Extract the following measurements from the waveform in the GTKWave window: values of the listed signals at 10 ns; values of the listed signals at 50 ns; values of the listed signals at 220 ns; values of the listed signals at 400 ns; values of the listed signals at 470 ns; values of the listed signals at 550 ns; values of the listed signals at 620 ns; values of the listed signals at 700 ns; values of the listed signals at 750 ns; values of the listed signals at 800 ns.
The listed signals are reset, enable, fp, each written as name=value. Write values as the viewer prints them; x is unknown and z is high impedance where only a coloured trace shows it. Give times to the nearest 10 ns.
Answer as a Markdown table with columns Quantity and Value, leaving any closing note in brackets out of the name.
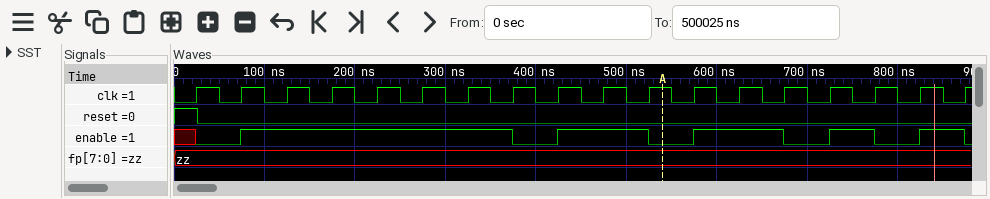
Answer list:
| Quantity | Value |
|---|---|
| values of the listed signals at 10 ns | reset=1, enable=x, fp=zz |
| values of the listed signals at 50 ns | reset=0, enable=0, fp=zz |
| values of the listed signals at 220 ns | reset=0, enable=1, fp=zz |
| values of the listed signals at 400 ns | reset=0, enable=0, fp=zz |
| values of the listed signals at 470 ns | reset=0, enable=1, fp=zz |
| values of the listed signals at 550 ns | reset=0, enable=0, fp=zz |
| values of the listed signals at 620 ns | reset=0, enable=1, fp=zz |
| values of the listed signals at 700 ns | reset=0, enable=0, fp=zz |
| values of the listed signals at 750 ns | reset=0, enable=1, fp=zz |
| values of the listed signals at 800 ns | reset=0, enable=0, fp=zz |
